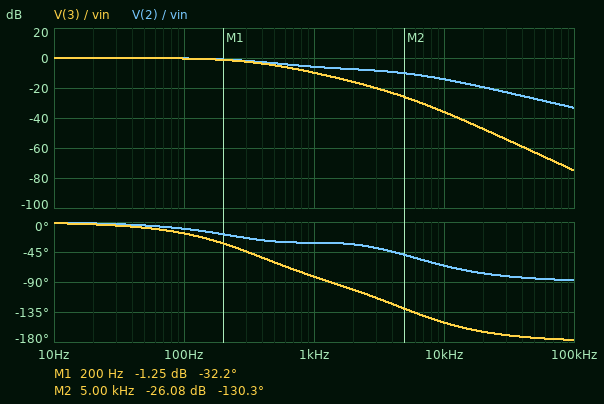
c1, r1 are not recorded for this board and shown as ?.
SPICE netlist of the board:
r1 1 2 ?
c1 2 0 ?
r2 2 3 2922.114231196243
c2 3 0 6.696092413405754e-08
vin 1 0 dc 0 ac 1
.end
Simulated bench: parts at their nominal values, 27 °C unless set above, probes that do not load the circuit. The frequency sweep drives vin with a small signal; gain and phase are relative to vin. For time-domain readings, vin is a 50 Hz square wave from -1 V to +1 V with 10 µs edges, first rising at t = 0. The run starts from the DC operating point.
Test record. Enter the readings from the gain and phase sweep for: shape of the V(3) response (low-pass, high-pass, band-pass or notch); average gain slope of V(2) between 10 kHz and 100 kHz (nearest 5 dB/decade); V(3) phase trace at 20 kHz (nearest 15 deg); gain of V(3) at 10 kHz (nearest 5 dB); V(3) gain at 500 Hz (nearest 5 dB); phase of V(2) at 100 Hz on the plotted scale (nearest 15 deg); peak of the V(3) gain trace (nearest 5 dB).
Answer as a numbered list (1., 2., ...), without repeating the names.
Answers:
1. low-pass
2. -20 dB/decade
3. -165 deg
4. -35 dB
5. -5 dB
6. -15 deg
7. 0 dB
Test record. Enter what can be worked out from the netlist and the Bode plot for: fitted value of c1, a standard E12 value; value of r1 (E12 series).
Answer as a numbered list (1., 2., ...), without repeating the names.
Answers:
1. 22 nF
2. 3.3 kΩ
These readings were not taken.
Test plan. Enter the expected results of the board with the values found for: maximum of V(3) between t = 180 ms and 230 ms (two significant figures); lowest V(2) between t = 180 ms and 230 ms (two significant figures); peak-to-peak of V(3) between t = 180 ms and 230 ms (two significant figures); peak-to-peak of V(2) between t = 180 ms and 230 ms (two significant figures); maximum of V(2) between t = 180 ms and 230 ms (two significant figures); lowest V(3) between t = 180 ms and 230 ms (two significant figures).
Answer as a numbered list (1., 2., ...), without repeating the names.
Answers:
1. 1.0 V
2. -1.0 V
3. 2.0 V
4. 2.0 V
5. 1.0 V
6. -1.0 V
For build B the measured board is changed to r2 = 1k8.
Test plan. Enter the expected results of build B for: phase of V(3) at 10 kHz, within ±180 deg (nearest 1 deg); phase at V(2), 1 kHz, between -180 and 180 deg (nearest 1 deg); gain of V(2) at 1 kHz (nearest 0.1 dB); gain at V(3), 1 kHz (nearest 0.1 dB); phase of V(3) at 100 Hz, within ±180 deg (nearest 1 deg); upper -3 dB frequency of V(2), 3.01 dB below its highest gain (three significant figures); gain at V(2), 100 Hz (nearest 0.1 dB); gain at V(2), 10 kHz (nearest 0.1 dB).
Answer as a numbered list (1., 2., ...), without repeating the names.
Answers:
1. -142 deg
2. -39 deg
3. -6.6 dB
4. -8.6 dB
5. -15 deg
6. 449 Hz
7. -0.2 dB
8. -14.9 dB
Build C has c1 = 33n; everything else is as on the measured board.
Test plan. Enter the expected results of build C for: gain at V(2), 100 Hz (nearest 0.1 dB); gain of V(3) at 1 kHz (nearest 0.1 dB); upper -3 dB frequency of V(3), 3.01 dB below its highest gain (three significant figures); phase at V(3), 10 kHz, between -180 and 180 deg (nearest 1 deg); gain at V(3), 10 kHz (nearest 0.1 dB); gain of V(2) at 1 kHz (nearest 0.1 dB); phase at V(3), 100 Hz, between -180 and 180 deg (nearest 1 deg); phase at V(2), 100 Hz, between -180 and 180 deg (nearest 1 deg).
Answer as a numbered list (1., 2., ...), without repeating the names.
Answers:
1. -0.3 dB
2. -10.4 dB
3. 328 Hz
4. -158 deg
5. -39.0 dB
6. -6.4 dB
7. -18 deg
8. -11 deg
